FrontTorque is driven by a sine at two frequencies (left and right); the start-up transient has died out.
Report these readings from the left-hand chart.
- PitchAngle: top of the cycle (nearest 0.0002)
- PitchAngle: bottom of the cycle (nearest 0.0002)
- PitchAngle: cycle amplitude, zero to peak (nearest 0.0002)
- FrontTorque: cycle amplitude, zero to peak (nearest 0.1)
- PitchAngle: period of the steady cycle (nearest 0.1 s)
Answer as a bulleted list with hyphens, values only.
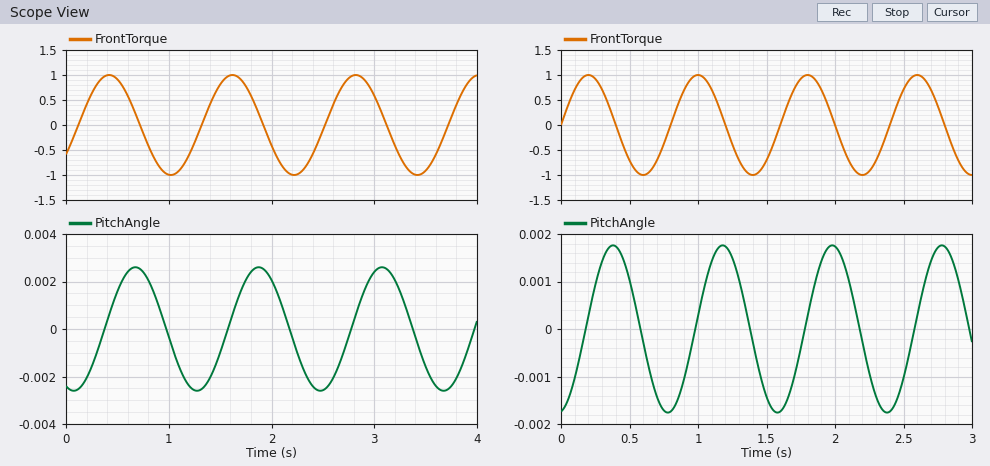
- 0.0026
- -0.0026
- 0.0026
- 1.0
- 1.2 s
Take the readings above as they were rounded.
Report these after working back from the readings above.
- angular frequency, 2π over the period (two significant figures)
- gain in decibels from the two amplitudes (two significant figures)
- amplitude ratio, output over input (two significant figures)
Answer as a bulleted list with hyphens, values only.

- 5.2 rad/s
- -52 dB
- 0.0026
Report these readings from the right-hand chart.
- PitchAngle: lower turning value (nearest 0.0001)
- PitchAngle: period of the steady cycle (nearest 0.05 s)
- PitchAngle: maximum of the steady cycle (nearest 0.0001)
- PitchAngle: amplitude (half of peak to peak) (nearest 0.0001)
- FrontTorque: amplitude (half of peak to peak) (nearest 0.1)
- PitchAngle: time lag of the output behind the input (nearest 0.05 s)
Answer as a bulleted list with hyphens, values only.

- -0.0018
- 0.80 s
- 0.0018
- 0.0018
- 1.0
- 0.20 s
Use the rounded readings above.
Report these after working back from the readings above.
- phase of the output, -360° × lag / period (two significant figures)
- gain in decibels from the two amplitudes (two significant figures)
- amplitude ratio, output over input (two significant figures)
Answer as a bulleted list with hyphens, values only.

- -90°
- -55 dB
- 0.0018
